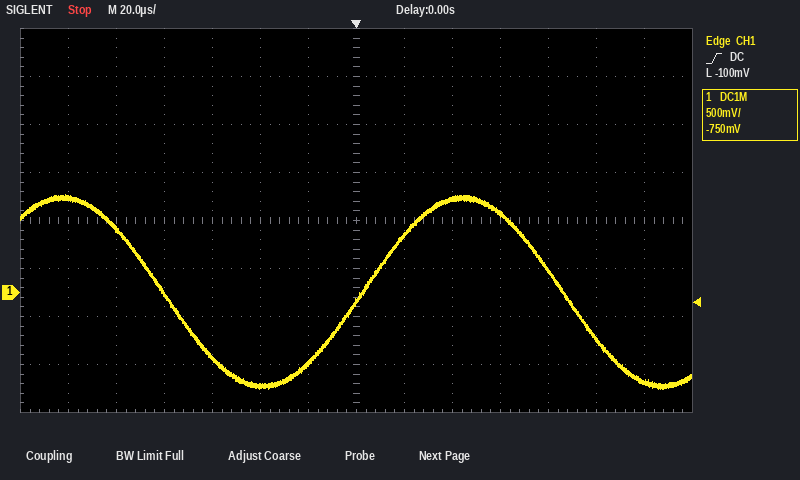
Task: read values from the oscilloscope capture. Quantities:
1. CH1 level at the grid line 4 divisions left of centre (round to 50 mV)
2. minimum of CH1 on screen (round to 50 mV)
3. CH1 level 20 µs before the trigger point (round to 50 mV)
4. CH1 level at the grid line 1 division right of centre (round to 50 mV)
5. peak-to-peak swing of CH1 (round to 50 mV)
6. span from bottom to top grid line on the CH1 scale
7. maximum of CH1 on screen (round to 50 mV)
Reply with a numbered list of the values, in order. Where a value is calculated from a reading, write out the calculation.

1. 0 mV
2. -1.00 V
3. -750 mV
4. 600 mV
5. 1.00 V − (-1.00 V) = 2.00 V
6. 4 V
7. 1.00 V
